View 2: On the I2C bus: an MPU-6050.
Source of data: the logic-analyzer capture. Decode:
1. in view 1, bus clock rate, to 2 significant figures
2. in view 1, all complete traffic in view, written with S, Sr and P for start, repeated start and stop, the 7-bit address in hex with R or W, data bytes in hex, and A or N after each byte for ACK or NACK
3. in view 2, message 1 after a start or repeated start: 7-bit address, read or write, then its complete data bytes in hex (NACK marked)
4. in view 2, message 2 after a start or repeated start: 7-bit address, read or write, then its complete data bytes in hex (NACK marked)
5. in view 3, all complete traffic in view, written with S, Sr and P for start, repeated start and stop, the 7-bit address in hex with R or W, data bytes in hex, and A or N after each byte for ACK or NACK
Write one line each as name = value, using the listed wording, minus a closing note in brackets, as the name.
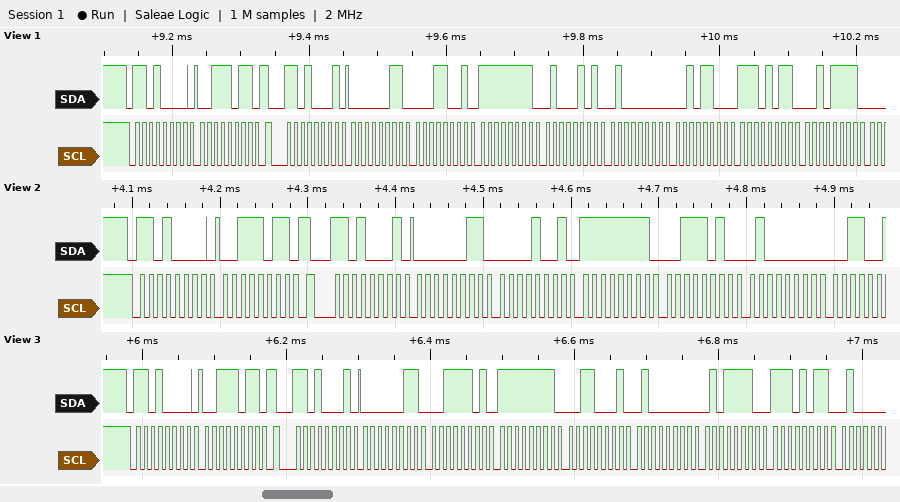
in view 1, bus clock rate, to 2 significant figures = 100 kHz
in view 1, all complete traffic in view, written with S, Sr and P for start, repeated start and stop, the 7-bit address in hex with R or W, data bytes in hex, and A or N after each byte for ACK or NACK = S 68W A 3B A Sr 68R A 03 A 19 A FF A 45 A 40 A 2C A EB A 2F A
in view 2, message 1 after a start or repeated start: 7-bit address, read or write, then its complete data bytes in hex = 0x68 write: 3B
in view 2, message 2 after a start or repeated start: 7-bit address, read or write, then its complete data bytes in hex = 0x68 read: 03 09 FF 3A 40
in view 3, all complete traffic in view, written with S, Sr and P for start, repeated start and stop, the 7-bit address in hex with R or W, data bytes in hex, and A or N after each byte for ACK or NACK = S 68W A 3B A Sr 68R A 03 A 3D A FF A 31 A 40 A 5E A EB A
